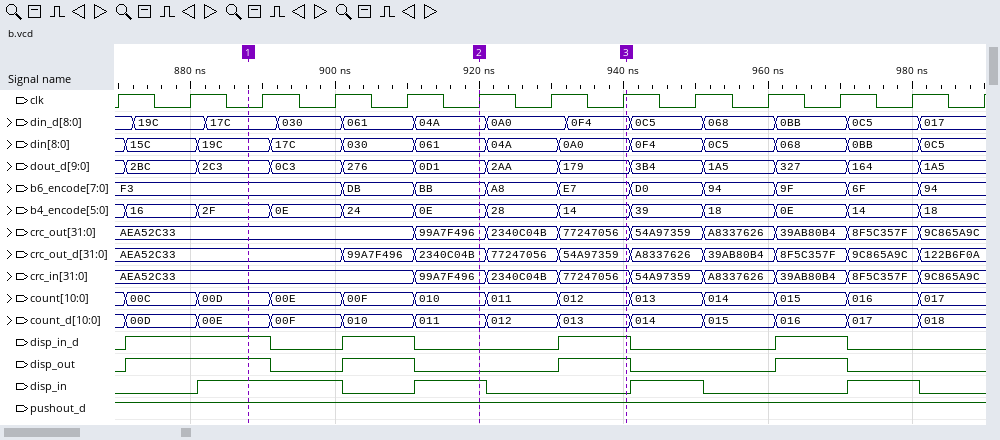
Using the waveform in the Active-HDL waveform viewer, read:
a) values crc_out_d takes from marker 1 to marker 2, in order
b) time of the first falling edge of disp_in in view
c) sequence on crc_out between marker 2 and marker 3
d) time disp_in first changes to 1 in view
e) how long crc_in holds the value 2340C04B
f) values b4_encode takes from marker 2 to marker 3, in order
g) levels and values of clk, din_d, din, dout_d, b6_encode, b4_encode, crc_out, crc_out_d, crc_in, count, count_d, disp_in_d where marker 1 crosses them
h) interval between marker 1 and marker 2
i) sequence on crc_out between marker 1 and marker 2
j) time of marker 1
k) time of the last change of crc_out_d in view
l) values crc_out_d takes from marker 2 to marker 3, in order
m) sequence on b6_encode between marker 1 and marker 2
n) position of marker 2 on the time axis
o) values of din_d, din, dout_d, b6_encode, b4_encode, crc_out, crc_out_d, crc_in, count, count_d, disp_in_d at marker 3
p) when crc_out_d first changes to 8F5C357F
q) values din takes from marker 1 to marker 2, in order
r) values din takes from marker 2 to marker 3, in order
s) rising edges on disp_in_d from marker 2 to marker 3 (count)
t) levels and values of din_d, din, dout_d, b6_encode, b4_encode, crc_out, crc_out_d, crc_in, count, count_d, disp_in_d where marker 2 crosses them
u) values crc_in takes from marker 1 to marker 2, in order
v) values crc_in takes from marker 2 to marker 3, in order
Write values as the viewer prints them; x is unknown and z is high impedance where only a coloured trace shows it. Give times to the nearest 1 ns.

AEA52C33, 99A7F496, 2340C04B
901 ns
99A7F496, 2340C04B, 77247056
881 ns
10 ns
0E, 28, 14
clk=0, din_d=17C, din=19C, dout_d=2C3, b6_encode=F3, b4_encode=2F, crc_out=AEA52C33, crc_out_d=AEA52C33, crc_in=AEA52C33, count=00D, count_d=00E, disp_in_d=1
32 ns
AEA52C33, 99A7F496
888 ns
981 ns
2340C04B, 77247056, 54A97359
F3, DB, BB
920 ns
din_d=0F4, din=0A0, dout_d=179, b6_encode=E7, b4_encode=14, crc_out=77247056, crc_out_d=54A97359, crc_in=77247056, count=012, count_d=013, disp_in_d=1
961 ns
19C, 17C, 030, 061
061, 04A, 0A0
1
din_d=04A, din=061, dout_d=0D1, b6_encode=BB, b4_encode=0E, crc_out=99A7F496, crc_out_d=2340C04B, crc_in=99A7F496, count=010, count_d=011, disp_in_d=0
AEA52C33, 99A7F496
99A7F496, 2340C04B, 77247056
